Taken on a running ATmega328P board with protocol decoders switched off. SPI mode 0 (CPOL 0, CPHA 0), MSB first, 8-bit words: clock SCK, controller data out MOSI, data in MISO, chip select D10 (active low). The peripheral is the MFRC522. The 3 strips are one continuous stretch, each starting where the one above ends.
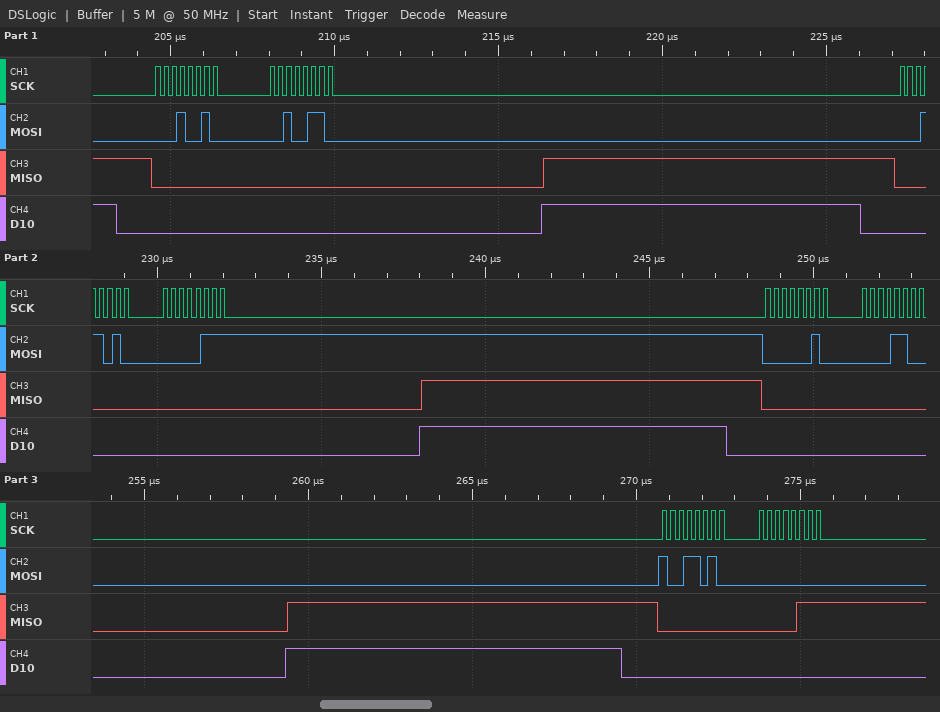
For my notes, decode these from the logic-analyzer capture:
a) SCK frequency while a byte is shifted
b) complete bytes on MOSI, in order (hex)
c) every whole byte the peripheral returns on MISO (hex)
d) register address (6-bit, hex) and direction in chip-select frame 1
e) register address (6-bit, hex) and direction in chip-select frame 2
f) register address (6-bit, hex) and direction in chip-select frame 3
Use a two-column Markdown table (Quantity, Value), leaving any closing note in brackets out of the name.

| Quantity | Value |
|---|---|
| SCK frequency while a byte is shifted | 4 MHz |
| complete bytes on MOSI, in order | 0x12 0x26 0x1A 0x07 0x02 0x0C 0x9A 0x00 |
| every whole byte the peripheral returns on MISO | 0x00 0x00 0x00 0x00 0x00 0x00 0x00 0x07 |
| register address (6-bit, hex) and direction in chip-select frame 1 | 0x09 write |
| register address (6-bit, hex) and direction in chip-select frame 2 | 0x0D write |
| register address (6-bit, hex) and direction in chip-select frame 3 | 0x01 write |
